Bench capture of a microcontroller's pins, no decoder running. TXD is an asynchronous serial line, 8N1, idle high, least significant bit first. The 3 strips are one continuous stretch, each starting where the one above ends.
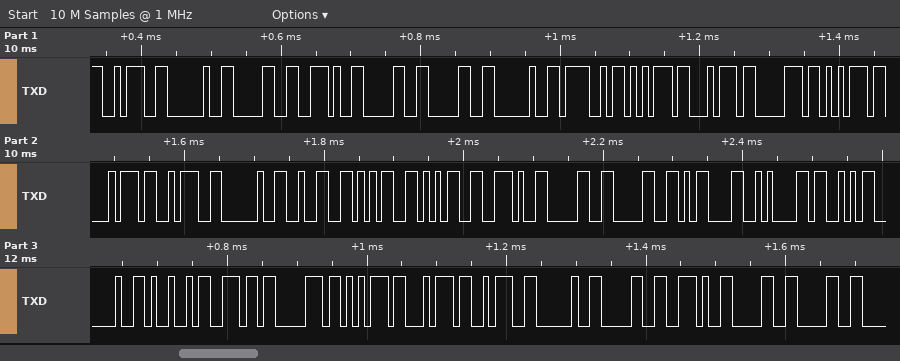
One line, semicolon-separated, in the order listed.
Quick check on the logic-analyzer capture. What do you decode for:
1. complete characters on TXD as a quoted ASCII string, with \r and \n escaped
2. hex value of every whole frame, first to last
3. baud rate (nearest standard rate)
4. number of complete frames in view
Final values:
": 0.00 Output: 255.00\r\nS Input: 0.00"; 0x3A 0x20 0x30 0x2E 0x30 0x30 0x20 0x4F 0x75 0x74 0x70 0x75 0x74 0x3A 0x20 0x32 0x35 0x35 0x2E 0x30 0x30 0x0D 0x0A 0x53 0x20 0x49 0x6E 0x70 0x75 0x74 0x3A 0x20 0x30 0x2E 0x30 0x30; 115200 baud; 36
